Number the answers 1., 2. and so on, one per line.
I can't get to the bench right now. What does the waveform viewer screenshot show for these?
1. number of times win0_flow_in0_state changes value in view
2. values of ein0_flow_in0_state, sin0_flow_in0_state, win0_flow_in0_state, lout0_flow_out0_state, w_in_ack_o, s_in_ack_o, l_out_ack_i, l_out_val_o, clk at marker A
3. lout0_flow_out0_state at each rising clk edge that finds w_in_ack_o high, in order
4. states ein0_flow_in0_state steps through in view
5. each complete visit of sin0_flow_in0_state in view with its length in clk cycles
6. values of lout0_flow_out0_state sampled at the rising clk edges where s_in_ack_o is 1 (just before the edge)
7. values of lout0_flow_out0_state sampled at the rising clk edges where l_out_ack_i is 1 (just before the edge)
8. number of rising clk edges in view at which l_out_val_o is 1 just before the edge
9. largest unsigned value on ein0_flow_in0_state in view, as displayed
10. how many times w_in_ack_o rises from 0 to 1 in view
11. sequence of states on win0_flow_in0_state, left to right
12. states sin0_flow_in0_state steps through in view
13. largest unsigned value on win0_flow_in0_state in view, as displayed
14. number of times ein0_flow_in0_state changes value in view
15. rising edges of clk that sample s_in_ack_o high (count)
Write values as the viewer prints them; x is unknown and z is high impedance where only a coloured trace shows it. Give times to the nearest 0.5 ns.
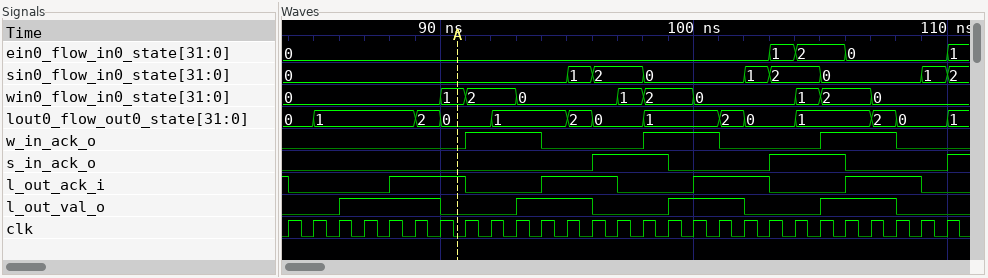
1. 9
2. ein0_flow_in0_state=0, sin0_flow_in0_state=0, win0_flow_in0_state=1, lout0_flow_out0_state=0, w_in_ack_o=0, s_in_ack_o=0, l_out_ack_i=1, l_out_val_o=0, clk=0
3. 0, 1, 1, 1, 1, 1, 1, 1, 2
4. 0, 1, 2, 0, 1
5. 1: 1, 2: 2, 0: 4, 1: 1, 2: 2, 0: 4, 1: 1
6. 0, 0, 1, 0, 1, 1
7. 0, 1, 2, 0, 1, 2, 0, 1, 2, 0, 1, 2, 0
8. 13
9. 2
10. 3
11. 0, 1, 2, 0, 1, 2, 0, 1, 2, 0
12. 0, 1, 2, 0, 1, 2, 0, 1, 2
13. 2
14. 4
15. 6
